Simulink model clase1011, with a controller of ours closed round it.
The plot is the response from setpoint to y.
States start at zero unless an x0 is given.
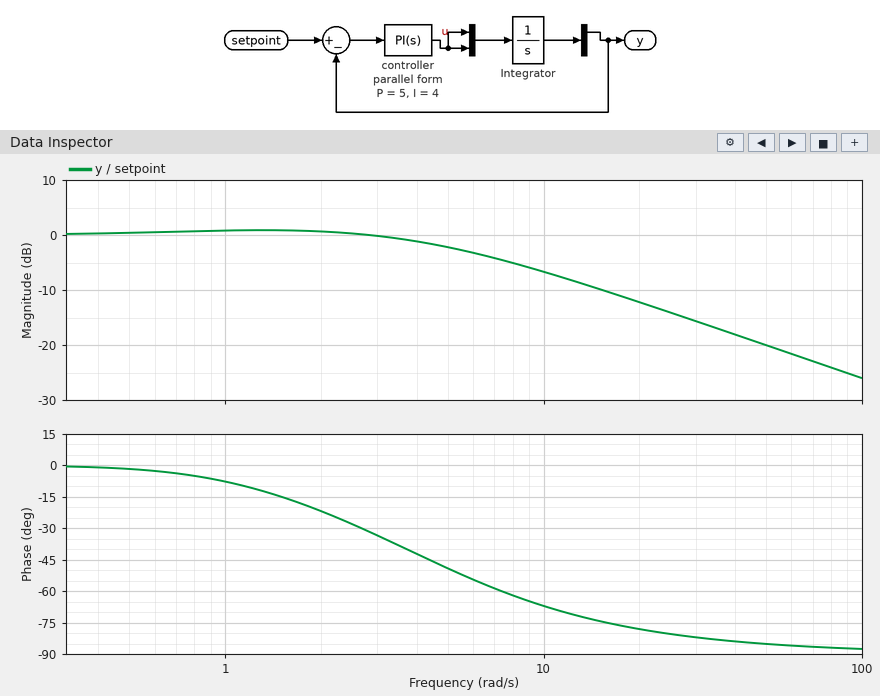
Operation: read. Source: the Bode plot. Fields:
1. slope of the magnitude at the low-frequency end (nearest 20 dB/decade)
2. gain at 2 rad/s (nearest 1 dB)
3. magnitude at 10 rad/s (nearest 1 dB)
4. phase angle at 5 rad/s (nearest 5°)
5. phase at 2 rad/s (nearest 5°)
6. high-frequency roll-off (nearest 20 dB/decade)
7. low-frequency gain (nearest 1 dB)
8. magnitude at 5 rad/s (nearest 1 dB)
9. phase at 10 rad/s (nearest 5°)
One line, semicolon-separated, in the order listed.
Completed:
0 dB/decade; 1 dB; -7 dB; -50°; -20°; -20 dB/decade; 0 dB; -2 dB; -65°
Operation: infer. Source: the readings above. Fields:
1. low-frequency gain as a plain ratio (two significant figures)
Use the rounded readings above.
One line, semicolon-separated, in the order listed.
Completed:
1.0
